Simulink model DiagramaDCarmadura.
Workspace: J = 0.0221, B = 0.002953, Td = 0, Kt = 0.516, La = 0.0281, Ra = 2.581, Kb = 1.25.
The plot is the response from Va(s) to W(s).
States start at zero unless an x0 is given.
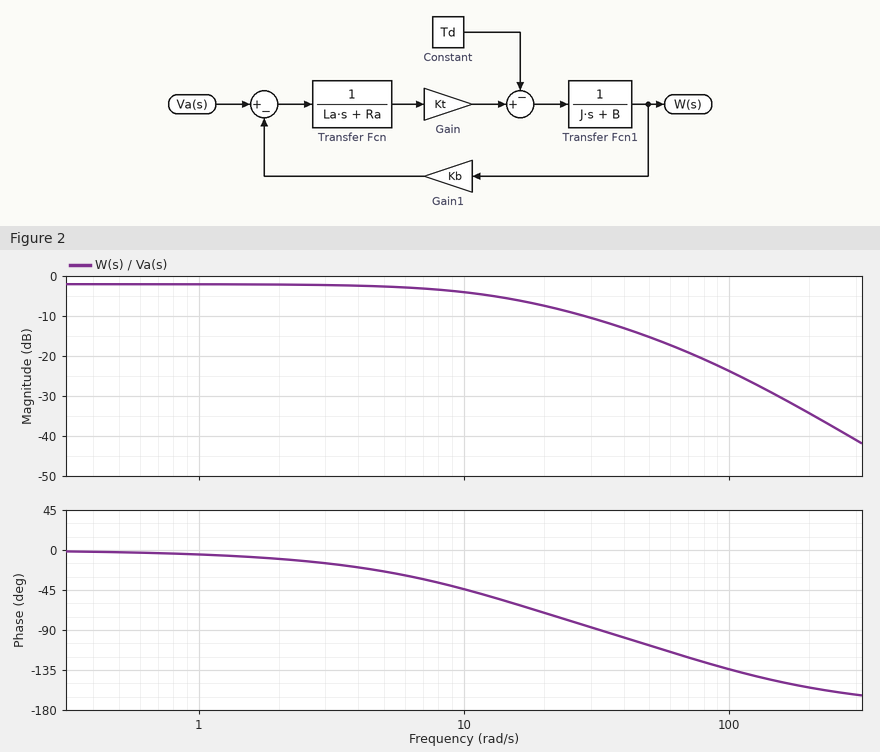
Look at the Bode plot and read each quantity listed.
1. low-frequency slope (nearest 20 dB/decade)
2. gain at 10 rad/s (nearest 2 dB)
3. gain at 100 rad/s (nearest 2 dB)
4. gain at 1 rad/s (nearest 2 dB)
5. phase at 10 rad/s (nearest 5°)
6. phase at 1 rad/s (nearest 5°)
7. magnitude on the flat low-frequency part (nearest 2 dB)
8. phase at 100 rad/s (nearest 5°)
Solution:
0 dB/decade
-4 dB
-24 dB
-2 dB
-45°
-5°
-2 dB
-135°
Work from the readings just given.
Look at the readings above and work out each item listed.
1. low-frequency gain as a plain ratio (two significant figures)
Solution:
0.79
